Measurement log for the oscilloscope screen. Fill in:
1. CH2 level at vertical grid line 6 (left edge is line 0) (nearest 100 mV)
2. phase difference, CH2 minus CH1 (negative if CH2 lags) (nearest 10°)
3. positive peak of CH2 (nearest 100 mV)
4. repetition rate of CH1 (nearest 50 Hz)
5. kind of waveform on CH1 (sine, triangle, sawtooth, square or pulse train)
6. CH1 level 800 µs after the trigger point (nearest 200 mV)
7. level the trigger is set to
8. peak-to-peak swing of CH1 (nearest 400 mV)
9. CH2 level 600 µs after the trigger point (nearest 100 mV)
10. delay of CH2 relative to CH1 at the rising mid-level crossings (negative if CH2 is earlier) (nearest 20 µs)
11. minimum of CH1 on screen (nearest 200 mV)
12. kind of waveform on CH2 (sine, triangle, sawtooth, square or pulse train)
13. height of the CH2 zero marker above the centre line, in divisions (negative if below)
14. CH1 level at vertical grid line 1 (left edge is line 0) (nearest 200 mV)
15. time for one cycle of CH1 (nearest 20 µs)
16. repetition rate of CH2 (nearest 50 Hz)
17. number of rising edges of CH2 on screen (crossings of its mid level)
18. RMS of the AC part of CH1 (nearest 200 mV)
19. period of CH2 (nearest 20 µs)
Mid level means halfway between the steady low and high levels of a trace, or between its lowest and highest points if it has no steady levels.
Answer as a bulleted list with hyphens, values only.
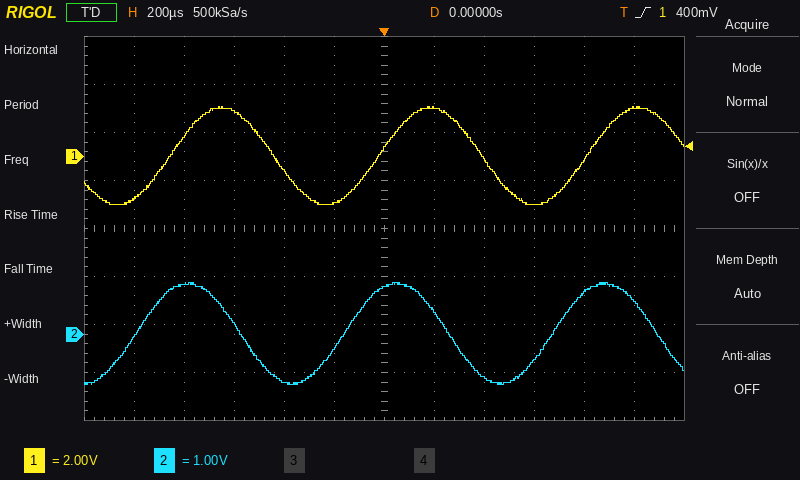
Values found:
- 1.0 V
- +60°
- 1.1 V
- 1.20 kHz
- sine
- -200 mV
- 400 mV
- 4.0 V
- -500 mV
- -140 µs
- -2.0 V
- sine
- -2.2 div
- -1.8 V
- 840 µs
- 1.20 kHz
- 3
- 1.4 V
- 840 µs
